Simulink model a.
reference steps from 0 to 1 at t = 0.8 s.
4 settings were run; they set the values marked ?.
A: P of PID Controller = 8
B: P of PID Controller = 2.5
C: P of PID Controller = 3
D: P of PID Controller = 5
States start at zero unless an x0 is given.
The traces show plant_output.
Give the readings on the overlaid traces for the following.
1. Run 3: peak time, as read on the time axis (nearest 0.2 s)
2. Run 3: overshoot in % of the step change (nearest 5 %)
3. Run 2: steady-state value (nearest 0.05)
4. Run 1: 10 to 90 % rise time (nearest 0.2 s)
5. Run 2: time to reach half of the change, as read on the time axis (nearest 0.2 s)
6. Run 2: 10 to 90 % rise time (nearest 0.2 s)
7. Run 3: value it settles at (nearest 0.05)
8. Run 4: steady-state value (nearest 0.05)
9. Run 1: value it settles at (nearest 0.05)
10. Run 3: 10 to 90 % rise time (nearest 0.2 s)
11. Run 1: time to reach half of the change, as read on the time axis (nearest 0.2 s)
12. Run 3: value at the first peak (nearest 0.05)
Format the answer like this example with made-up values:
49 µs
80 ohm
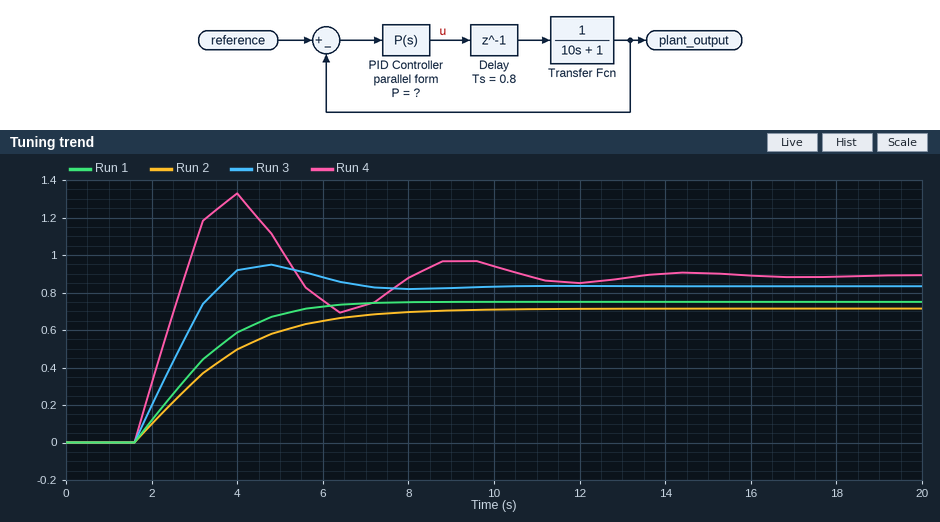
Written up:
4.8 s
15 %
0.70
3.0 s
3.2 s
4.0 s
0.85
0.90
0.75
1.4 s
3.0 s
0.95
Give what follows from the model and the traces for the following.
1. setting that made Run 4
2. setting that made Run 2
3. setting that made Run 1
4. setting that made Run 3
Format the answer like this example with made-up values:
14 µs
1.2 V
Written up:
A
B
C
D
